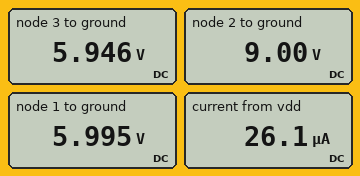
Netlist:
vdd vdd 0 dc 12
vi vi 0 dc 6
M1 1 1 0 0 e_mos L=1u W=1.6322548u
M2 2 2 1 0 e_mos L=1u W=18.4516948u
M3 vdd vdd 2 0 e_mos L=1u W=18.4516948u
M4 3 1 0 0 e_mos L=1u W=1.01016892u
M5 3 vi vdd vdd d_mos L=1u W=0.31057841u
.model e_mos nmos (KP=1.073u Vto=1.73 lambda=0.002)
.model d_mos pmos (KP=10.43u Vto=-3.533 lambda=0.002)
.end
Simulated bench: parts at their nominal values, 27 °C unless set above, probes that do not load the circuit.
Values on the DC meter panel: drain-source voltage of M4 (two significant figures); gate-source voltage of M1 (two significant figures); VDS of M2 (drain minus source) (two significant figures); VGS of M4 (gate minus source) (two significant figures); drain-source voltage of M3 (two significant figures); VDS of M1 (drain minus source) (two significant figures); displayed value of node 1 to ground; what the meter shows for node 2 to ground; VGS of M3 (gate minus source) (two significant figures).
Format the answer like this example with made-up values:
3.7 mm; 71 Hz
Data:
5.9 V; 6.0 V; 3.0 V; 6.0 V; 3.0 V; 6.0 V; 5.995 V; 9.00 V; 3.0 V
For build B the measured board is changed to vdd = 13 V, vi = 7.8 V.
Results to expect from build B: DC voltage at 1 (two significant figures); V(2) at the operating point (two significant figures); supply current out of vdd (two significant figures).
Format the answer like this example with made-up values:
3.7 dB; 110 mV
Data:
6.6 V; 9.8 V; 26 µA
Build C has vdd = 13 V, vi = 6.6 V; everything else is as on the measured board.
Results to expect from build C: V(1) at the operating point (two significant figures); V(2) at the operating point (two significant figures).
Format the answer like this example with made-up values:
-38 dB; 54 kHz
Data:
6.6 V; 9.8 V
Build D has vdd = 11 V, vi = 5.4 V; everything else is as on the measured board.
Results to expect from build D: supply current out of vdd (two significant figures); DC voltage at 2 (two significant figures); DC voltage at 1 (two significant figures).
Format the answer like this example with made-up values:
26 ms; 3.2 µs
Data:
19 µA; 8.2 V; 5.4 V
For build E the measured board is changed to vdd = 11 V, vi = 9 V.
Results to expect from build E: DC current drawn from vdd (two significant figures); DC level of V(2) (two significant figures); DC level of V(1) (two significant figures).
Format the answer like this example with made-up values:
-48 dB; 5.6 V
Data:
12 µA; 8.2 V; 5.4 V
